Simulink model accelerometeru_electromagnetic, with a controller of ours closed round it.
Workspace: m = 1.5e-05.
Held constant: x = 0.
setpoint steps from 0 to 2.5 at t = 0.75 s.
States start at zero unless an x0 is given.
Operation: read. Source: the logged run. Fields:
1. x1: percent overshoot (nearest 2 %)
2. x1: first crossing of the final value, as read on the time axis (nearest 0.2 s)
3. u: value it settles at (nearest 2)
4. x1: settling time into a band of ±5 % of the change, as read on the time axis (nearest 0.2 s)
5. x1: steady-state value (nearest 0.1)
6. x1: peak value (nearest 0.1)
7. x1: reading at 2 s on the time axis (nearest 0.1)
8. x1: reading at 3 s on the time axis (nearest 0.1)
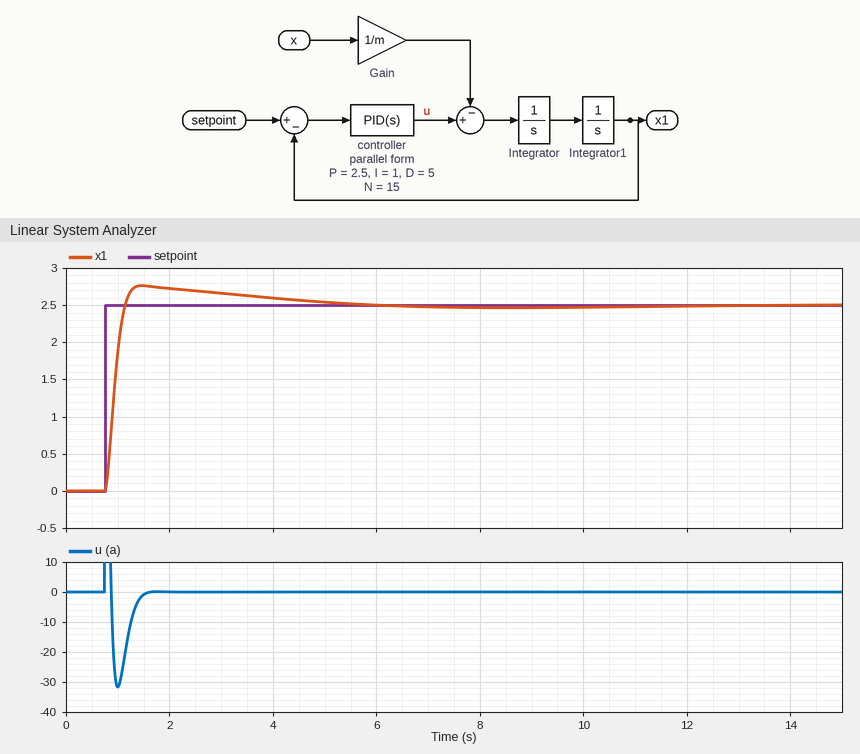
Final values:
10 %
1.2 s
0
3.6 s
2.5
2.8
2.7
2.7
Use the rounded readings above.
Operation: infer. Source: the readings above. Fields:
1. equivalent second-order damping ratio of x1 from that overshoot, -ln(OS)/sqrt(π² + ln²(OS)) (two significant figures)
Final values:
0.59
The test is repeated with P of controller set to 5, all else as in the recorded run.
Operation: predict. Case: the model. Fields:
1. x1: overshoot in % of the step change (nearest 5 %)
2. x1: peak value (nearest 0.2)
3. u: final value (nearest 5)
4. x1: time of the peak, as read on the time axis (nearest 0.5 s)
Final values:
15 %
3.0
0
1.5 s
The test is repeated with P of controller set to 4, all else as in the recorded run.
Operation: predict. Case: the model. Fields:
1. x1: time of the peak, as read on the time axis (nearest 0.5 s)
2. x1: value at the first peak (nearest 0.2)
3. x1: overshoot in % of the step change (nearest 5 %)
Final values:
1.5 s
2.8
15 %
